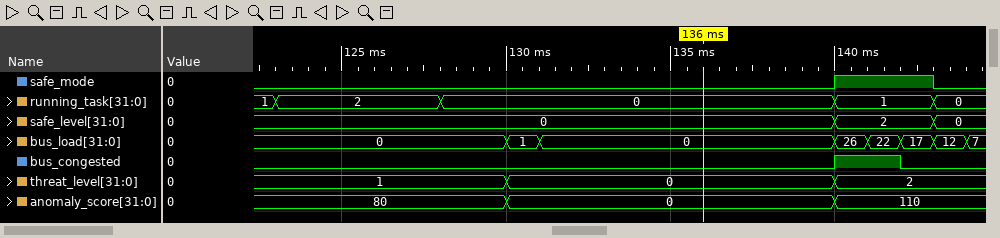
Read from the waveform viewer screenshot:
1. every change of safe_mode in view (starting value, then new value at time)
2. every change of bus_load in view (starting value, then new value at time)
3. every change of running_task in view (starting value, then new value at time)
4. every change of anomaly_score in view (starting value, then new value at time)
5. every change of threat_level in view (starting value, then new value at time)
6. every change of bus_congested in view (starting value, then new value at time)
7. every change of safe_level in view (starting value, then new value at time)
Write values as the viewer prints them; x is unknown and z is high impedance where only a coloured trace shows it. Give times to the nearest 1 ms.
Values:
0, 1 at 140 ms, 0 at 143 ms
0, 1 at 130 ms, 0 at 131 ms, 26 at 140 ms, 22 at 141 ms, 17 at 142 ms, 12 at 143 ms, 7 at 144 ms
1, 2 at 123 ms, 0 at 128 ms, 1 at 140 ms, 0 at 143 ms
80, 0 at 130 ms, 110 at 140 ms
1, 0 at 130 ms, 2 at 140 ms
0, 1 at 140 ms, 0 at 142 ms
0, 2 at 140 ms, 0 at 143 ms
